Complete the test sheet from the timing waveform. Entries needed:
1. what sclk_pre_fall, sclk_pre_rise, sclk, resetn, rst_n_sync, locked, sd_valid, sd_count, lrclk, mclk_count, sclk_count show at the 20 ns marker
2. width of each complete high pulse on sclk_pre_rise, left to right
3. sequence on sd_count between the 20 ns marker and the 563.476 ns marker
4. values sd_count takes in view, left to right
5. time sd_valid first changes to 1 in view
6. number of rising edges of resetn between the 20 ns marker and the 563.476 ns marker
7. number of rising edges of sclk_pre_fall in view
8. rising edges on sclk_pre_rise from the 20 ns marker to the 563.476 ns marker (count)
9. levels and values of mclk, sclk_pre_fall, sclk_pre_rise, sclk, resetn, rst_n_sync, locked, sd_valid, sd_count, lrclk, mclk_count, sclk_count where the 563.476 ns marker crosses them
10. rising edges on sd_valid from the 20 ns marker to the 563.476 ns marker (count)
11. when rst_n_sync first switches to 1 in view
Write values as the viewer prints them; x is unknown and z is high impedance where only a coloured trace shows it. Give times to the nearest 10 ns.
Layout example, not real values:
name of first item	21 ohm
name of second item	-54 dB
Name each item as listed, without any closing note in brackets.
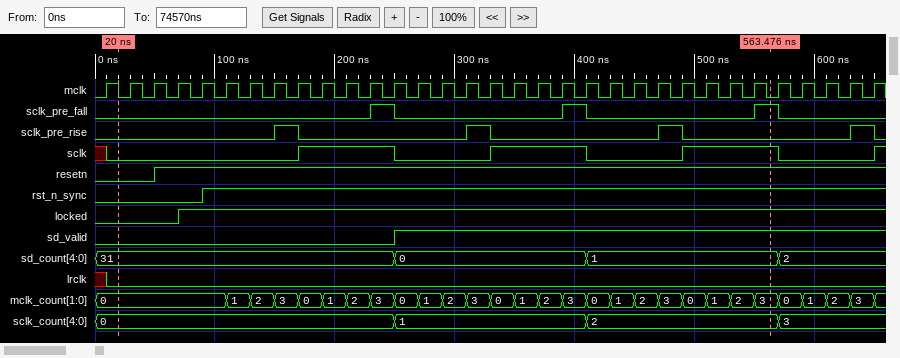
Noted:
what sclk_pre_fall, sclk_pre_rise, sclk, resetn, rst_n_sync, locked, sd_valid, sd_count, lrclk, mclk_count, sclk_count show at the 20 ns marker	sclk_pre_fall=0, sclk_pre_rise=0, sclk=0, resetn=0, rst_n_sync=0, locked=0, sd_valid=0, sd_count=31, lrclk=0, mclk_count=0, sclk_count=0
width of each complete high pulse on sclk_pre_rise, left to right	20 ns, 20 ns, 20 ns, 20 ns
sequence on sd_count between the 20 ns marker and the 563.476 ns marker	31, 0, 1
values sd_count takes in view, left to right	31, 0, 1, 2
time sd_valid first changes to 1 in view	250 ns
number of rising edges of resetn between the 20 ns marker and the 563.476 ns marker	1
number of rising edges of sclk_pre_fall in view	3
rising edges on sclk_pre_rise from the 20 ns marker to the 563.476 ns marker	3
levels and values of mclk, sclk_pre_fall, sclk_pre_rise, sclk, resetn, rst_n_sync, locked, sd_valid, sd_count, lrclk, mclk_count, sclk_count where the 563.476 ns marker crosses them	mclk=0, sclk_pre_fall=1, sclk_pre_rise=0, sclk=1, resetn=1, rst_n_sync=1, locked=1, sd_valid=1, sd_count=1, lrclk=0, mclk_count=3, sclk_count=2
rising edges on sd_valid from the 20 ns marker to the 563.476 ns marker	1
when rst_n_sync first switches to 1 in view	90 ns
